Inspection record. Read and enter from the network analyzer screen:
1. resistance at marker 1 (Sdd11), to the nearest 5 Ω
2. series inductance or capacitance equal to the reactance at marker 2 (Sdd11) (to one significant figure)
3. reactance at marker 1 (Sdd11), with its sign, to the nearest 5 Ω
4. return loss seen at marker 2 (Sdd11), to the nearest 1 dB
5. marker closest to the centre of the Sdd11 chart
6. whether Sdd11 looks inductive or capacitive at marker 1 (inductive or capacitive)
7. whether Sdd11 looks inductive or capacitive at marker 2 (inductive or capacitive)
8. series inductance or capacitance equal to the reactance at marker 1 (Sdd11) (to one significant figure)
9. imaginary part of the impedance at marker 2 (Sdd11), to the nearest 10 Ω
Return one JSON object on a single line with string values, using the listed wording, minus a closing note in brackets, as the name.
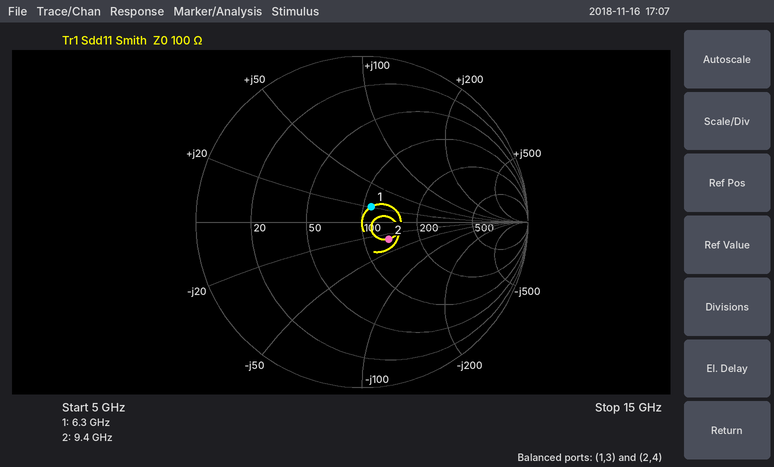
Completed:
{"resistance at marker 1 (Sdd11), to the nearest 5 Ω": "110 Ω", "series inductance or capacitance equal to the reactance at marker 2 (Sdd11)": "600 fF", "reactance at marker 1 (Sdd11), with its sign, to the nearest 5 Ω": "+20 Ω", "return loss seen at marker 2 (Sdd11), to the nearest 1 dB": "14 dB", "marker closest to the centre of the Sdd11 chart": "marker 1", "whether Sdd11 looks inductive or capacitive at marker 1": "inductive", "whether Sdd11 looks inductive or capacitive at marker 2": "capacitive", "series inductance or capacitance equal to the reactance at marker 1 (Sdd11)": "500 pH", "imaginary part of the impedance at marker 2 (Sdd11), to the nearest 10 Ω": "-30 Ω"}
